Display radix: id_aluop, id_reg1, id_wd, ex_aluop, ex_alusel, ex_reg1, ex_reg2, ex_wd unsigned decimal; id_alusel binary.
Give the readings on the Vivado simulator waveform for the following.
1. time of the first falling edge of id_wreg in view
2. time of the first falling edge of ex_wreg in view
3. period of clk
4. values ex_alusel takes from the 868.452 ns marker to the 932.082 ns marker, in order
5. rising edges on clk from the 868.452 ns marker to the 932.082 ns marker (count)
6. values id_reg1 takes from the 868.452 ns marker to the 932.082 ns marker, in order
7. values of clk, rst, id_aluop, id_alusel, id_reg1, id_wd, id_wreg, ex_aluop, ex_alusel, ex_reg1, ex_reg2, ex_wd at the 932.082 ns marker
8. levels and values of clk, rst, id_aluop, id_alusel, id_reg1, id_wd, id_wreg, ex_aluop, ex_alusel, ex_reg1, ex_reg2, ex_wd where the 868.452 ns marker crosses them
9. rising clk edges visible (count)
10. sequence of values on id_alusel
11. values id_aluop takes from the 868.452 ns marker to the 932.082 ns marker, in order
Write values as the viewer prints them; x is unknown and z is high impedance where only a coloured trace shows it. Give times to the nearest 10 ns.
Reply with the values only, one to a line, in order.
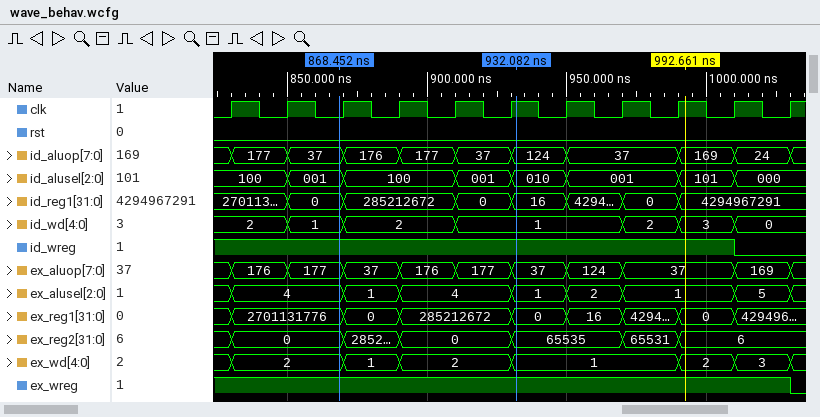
1010 ns
1030 ns
20 ns
4, 1, 4, 1
4
0, 285212672, 0, 16
clk=1, rst=0, id_aluop=124, id_alusel=010, id_reg1=16, id_wd=1, id_wreg=1, ex_aluop=37, ex_alusel=1, ex_reg1=0, ex_reg2=65535, ex_wd=1
clk=0, rst=0, id_aluop=37, id_alusel=001, id_reg1=0, id_wd=1, id_wreg=1, ex_aluop=177, ex_alusel=4, ex_reg1=2701131776, ex_reg2=0, ex_wd=2
11
100, 001, 100, 001, 010, 001, 101, 000
37, 176, 177, 37, 124
